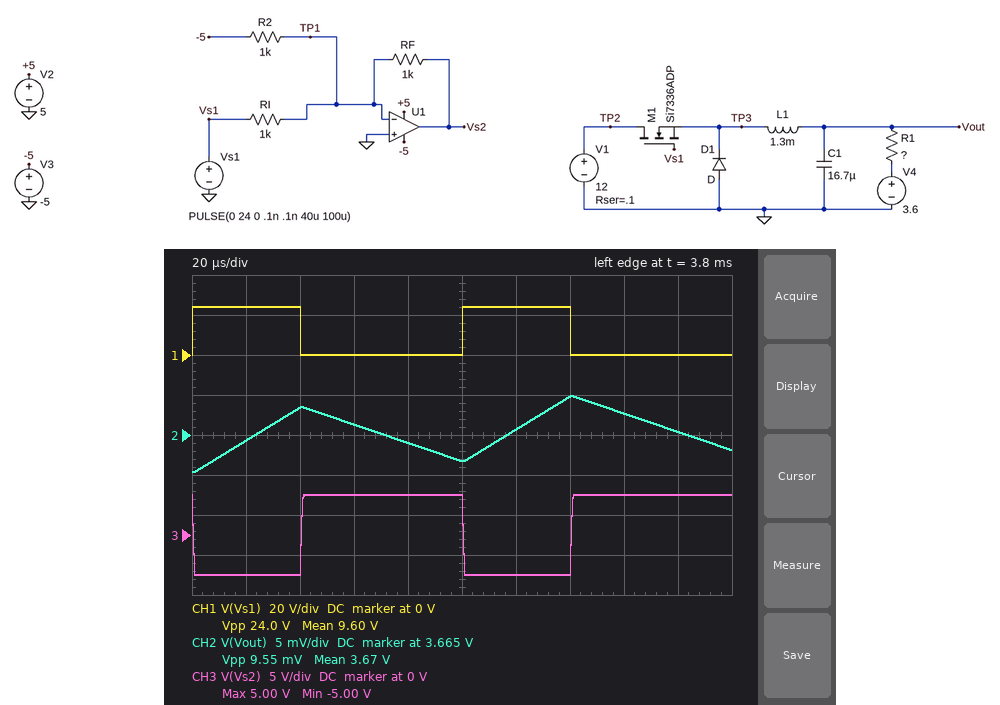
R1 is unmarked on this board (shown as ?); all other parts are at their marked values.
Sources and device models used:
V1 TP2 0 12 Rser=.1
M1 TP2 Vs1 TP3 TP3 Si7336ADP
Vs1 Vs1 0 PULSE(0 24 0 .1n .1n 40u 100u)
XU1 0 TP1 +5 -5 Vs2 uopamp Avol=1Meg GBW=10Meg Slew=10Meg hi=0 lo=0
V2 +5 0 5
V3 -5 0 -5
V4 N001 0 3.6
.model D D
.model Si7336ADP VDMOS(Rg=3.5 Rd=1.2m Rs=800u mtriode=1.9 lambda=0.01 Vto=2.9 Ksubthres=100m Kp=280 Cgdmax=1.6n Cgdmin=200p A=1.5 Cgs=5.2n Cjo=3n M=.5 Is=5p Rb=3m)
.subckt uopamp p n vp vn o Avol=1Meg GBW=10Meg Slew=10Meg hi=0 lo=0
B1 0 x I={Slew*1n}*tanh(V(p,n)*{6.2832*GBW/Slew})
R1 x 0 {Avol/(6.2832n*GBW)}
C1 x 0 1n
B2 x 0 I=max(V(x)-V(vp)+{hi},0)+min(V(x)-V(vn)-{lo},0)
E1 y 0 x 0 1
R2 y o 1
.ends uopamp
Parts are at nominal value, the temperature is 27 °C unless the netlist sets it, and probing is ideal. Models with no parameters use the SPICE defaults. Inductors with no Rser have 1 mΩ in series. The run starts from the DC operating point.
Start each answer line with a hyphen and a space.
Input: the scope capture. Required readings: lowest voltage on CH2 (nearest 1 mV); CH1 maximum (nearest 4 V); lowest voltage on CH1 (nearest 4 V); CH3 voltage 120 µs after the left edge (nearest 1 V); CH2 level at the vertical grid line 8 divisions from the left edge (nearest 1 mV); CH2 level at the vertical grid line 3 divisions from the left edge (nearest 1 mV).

- 3.660 V
- 24 V
- 0 V
- -5 V
- 3.668 V
- 3.666 V
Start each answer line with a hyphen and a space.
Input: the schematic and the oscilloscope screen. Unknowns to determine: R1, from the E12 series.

- 0.033 Ω
